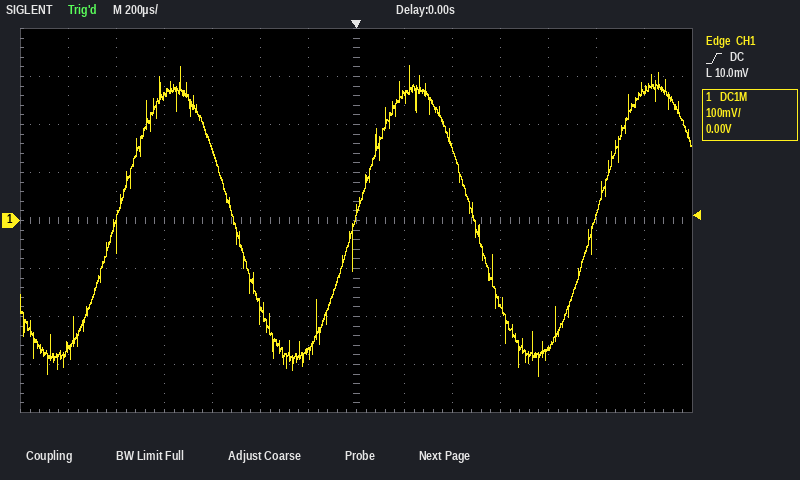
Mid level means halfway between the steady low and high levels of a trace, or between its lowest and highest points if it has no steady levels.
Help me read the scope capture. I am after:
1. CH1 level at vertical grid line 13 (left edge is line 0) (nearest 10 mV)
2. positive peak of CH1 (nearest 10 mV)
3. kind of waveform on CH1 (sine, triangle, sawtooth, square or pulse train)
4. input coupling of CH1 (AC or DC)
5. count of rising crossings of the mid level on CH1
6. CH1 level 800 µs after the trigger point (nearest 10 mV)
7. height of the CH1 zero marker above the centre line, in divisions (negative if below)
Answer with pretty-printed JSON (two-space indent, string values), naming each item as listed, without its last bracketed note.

{
  "CH1 level at vertical grid line 13 (left edge is line 0)": "270 mV",
  "positive peak of CH1": "320 mV",
  "kind of waveform on CH1": "sine",
  "input coupling of CH1": "DC",
  "count of rising crossings of the mid level on CH1": "3",
  "CH1 level 800 µs after the trigger point": "-270 mV",
  "height of the CH1 zero marker above the centre line, in divisions": "0.0 div"
}
